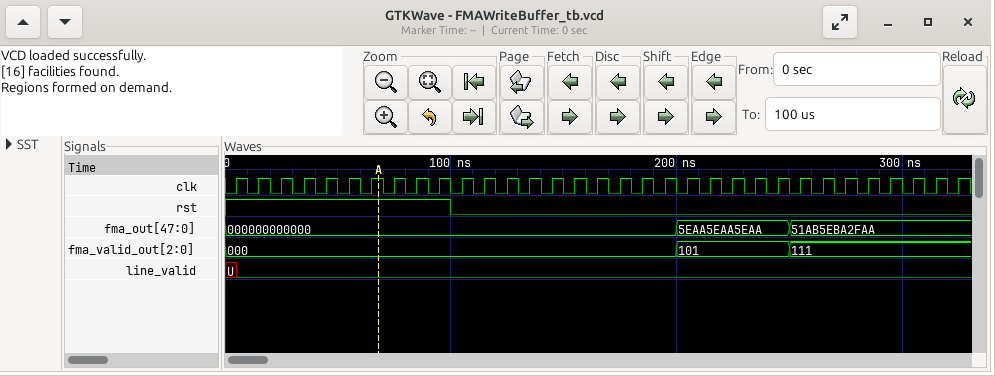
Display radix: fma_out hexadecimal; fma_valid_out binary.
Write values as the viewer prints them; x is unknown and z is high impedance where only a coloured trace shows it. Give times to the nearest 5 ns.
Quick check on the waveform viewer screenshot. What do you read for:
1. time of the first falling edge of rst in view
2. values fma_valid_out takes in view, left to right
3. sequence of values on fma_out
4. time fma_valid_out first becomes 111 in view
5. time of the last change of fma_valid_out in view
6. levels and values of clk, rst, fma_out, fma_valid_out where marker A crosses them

100 ns
000, 101, 111
000000000000, 5EAA5EAA5EAA, 51AB5EBA2FAA
250 ns
250 ns
clk=1, rst=1, fma_out=000000000000, fma_valid_out=000
